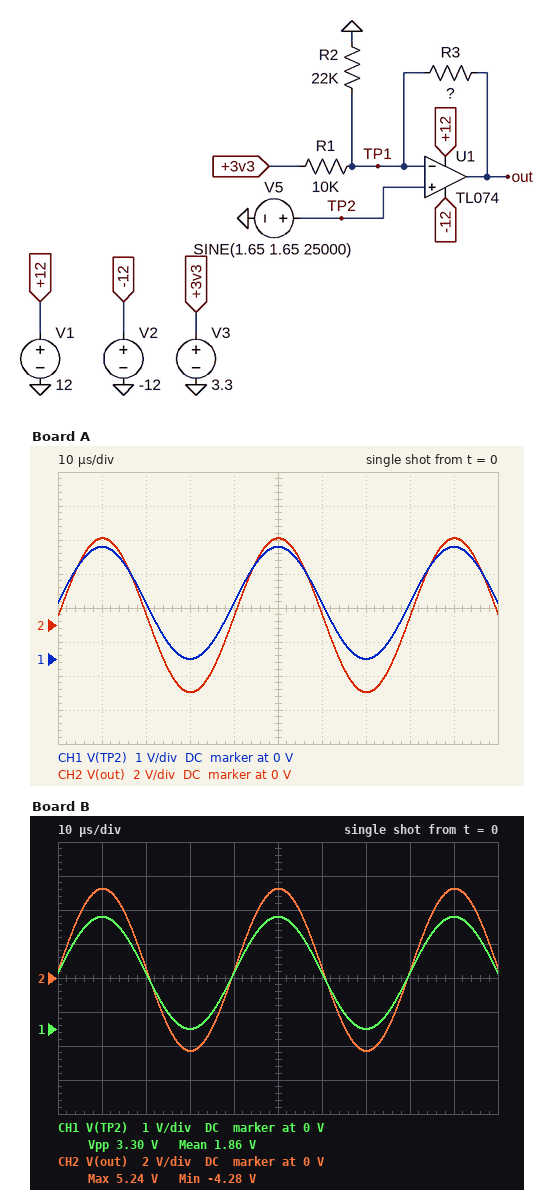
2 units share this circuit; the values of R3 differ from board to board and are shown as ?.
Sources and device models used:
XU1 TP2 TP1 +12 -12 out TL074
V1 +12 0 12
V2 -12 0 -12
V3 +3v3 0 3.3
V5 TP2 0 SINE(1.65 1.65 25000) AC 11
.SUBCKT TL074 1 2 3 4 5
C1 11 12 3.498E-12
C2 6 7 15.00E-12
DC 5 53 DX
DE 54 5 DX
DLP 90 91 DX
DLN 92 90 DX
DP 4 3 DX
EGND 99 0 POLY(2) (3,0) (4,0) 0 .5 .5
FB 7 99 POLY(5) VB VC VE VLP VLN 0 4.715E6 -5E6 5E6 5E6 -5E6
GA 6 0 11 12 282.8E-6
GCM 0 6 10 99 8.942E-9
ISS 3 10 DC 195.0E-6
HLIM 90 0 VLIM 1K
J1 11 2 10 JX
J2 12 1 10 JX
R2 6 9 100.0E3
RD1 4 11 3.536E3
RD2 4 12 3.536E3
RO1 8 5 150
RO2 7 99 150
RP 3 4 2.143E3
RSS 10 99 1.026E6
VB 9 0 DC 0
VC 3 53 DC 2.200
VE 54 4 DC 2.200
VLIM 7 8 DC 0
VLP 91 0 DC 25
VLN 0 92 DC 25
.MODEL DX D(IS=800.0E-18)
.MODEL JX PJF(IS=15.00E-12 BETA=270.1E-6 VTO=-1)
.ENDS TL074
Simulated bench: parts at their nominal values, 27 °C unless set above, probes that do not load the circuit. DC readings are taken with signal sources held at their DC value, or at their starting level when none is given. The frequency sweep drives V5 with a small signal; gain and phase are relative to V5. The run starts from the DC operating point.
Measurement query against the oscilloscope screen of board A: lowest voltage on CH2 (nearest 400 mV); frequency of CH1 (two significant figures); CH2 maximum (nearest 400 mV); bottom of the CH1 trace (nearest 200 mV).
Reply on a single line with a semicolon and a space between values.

-4.0 V; 25 kHz; 5.2 V; 0 V
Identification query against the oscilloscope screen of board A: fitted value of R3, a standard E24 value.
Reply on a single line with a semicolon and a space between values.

12 kΩ
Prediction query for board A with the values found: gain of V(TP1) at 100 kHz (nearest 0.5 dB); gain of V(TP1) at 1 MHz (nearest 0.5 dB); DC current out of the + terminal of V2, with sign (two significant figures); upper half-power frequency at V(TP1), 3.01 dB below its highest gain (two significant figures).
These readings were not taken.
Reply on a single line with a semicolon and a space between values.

0 dB; -1.5 dB; -11 mA; 1.5 MHz
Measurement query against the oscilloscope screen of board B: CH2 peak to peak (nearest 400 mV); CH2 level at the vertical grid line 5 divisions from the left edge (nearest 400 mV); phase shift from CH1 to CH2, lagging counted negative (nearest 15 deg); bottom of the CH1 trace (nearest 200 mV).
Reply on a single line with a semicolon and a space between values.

9.6 V; 5.2 V; 0 deg; 0 V
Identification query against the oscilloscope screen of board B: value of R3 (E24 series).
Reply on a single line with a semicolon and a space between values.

13 kΩ
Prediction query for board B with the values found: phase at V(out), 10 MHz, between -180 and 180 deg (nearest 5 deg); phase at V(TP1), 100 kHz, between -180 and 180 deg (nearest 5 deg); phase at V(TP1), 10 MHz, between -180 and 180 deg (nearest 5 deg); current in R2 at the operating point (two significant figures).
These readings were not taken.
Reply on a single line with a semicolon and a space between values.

-145 deg; -5 deg; -145 deg; 75 µA
